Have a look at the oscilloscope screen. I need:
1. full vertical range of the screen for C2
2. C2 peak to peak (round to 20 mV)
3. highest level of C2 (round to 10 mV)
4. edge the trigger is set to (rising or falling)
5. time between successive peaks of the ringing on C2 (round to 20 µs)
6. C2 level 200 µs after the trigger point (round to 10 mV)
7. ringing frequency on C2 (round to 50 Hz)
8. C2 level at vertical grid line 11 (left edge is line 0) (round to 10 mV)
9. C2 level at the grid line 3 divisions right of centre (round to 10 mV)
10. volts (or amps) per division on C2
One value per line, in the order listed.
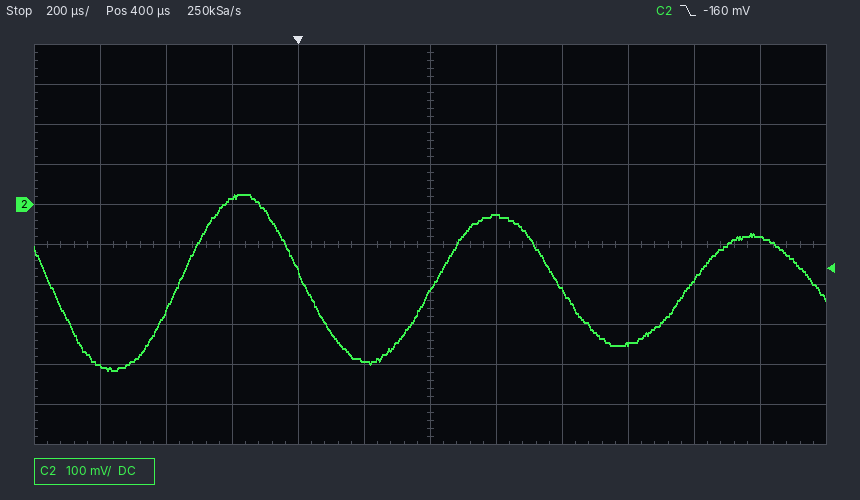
1 V
440 mV
20 mV
falling
780 µs
-390 mV
1.30 kHz
-80 mV
-350 mV
100 mV
